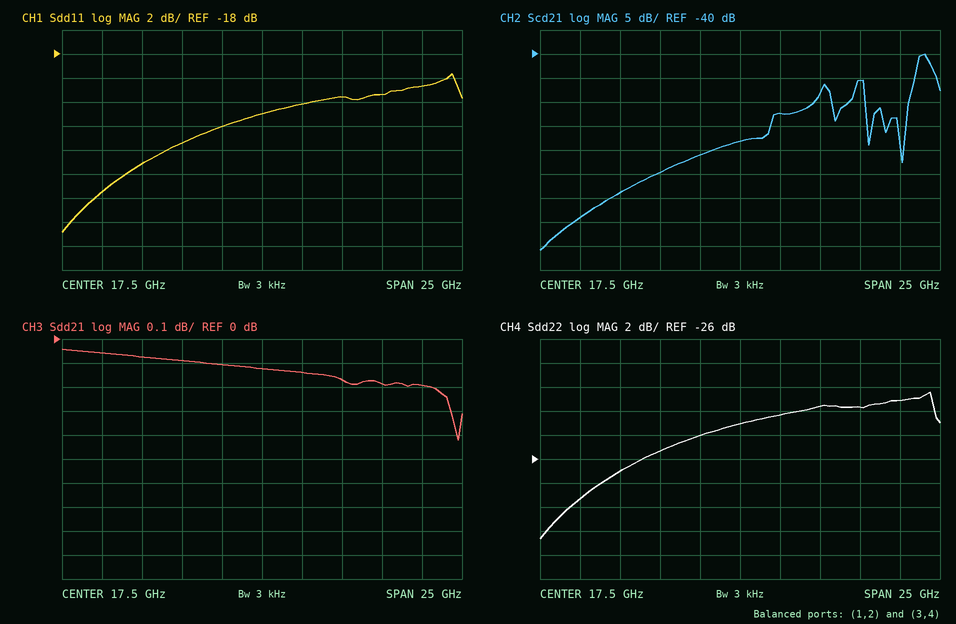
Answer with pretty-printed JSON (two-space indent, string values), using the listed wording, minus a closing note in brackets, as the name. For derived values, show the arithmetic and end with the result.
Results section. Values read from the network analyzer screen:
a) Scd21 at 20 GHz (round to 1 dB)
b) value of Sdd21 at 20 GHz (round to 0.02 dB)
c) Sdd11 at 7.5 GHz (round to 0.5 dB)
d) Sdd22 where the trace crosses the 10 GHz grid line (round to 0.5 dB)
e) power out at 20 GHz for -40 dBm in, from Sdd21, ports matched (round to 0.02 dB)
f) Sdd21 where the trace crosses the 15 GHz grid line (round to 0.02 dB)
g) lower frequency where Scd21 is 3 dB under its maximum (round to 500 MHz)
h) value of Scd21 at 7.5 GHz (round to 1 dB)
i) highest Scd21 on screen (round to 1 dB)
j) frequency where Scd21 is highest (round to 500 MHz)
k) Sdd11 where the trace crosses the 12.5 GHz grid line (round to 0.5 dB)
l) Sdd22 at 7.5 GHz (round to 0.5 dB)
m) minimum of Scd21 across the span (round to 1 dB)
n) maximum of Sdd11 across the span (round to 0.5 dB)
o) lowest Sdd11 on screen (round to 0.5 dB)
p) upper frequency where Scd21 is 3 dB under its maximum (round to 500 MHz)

{
  "Scd21 at 20 GHz": "-52 dB",
  "value of Sdd21 at 20 GHz": "-0.14 dB",
  "Sdd11 at 7.5 GHz": "-29.5 dB",
  "Sdd22 where the trace crosses the 10 GHz grid line": "-27.0 dB",
  "power out at 20 GHz for -40 dBm in, from Sdd21, ports matched": "-40 dBm + (-0.14 dB) = -40.14 dBm",
  "Sdd21 where the trace crosses the 15 GHz grid line": "-0.10 dB",
  "lower frequency where Scd21 is 3 dB under its maximum": "28.5 GHz",
  "value of Scd21 at 7.5 GHz": "-74 dB",
  "highest Scd21 on screen": "-40 dB",
  "frequency where Scd21 is highest": "29.0 GHz",
  "Sdd11 where the trace crosses the 12.5 GHz grid line": "-25.5 dB",
  "Sdd22 at 7.5 GHz": "-29.5 dB",
  "minimum of Scd21 across the span": "-81 dB",
  "maximum of Sdd11 across the span": "-19.5 dB",
  "lowest Sdd11 on screen": "-33.0 dB",
  "upper frequency where Scd21 is 3 dB under its maximum": "29.5 GHz"
}
